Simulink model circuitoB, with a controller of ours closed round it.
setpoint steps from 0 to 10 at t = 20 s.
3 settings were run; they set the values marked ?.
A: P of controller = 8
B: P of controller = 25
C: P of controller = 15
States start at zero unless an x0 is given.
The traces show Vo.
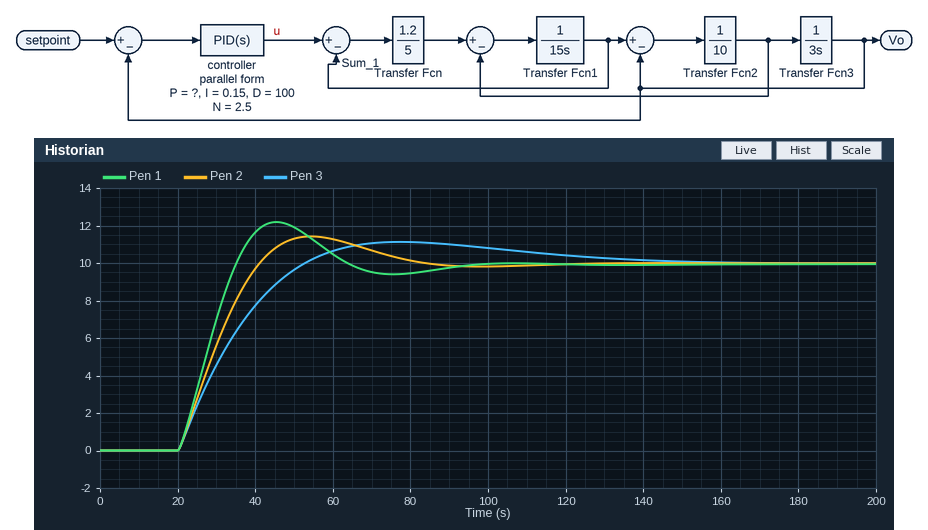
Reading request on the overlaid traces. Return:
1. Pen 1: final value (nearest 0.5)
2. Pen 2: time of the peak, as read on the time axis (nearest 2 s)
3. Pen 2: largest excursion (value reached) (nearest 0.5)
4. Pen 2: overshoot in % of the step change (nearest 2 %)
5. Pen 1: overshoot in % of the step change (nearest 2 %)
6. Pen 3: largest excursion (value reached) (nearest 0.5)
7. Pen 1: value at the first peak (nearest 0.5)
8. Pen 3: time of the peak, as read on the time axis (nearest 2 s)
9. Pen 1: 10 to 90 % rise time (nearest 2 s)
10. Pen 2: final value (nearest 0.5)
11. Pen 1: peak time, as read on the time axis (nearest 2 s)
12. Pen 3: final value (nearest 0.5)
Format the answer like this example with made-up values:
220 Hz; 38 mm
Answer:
10.0; 54 s; 11.5; 14 %; 22 %; 11.0; 12.0; 78 s; 12 s; 10.0; 46 s; 10.0
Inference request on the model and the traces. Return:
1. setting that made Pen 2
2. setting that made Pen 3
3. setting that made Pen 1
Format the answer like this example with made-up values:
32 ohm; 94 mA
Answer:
C; A; B
